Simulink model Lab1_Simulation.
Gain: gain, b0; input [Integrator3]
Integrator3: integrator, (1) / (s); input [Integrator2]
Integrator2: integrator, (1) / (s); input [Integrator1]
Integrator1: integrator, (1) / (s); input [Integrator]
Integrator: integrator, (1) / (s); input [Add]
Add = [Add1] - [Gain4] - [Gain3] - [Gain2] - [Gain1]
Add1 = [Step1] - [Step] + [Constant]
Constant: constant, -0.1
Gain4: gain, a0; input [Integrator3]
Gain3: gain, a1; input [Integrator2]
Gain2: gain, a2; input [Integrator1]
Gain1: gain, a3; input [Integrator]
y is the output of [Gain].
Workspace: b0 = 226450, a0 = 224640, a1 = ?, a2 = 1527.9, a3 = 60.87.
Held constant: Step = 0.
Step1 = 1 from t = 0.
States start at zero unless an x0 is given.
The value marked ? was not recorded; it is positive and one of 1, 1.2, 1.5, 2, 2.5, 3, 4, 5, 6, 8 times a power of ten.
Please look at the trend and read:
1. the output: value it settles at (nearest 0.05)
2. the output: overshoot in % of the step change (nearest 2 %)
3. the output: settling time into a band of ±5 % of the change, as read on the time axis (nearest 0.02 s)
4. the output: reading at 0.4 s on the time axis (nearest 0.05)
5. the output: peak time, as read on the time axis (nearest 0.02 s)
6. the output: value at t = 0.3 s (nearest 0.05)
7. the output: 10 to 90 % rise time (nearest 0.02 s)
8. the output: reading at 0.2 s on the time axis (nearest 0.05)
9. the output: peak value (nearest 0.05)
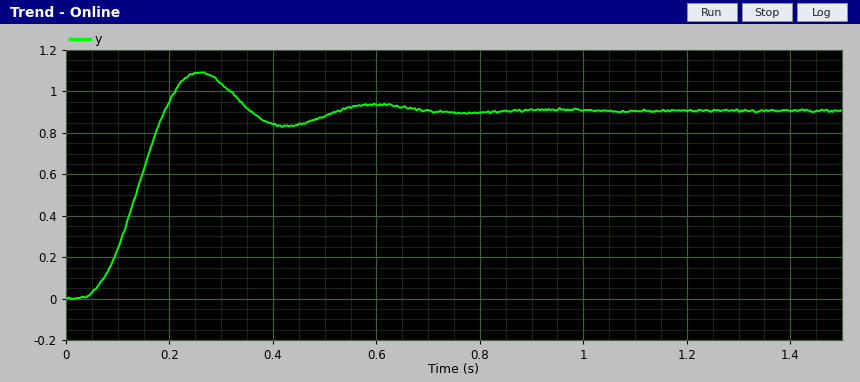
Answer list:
0.90
20 %
0.48 s
0.85
0.26 s
1.05
0.10 s
0.95
1.10
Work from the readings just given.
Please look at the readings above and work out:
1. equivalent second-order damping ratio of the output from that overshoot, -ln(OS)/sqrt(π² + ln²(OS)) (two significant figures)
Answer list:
0.46
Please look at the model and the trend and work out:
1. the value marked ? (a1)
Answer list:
25000
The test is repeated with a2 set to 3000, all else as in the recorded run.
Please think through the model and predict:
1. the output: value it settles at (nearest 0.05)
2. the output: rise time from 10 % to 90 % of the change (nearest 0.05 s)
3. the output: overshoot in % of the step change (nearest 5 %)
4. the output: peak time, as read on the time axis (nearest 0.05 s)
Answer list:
0.90
0.15 s
25 %
0.40 s
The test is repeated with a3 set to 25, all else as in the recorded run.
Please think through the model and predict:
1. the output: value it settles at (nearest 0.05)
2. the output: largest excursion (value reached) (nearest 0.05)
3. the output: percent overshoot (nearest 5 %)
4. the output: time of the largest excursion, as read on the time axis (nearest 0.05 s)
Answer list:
0.90
1.00
10 %
0.35 s
